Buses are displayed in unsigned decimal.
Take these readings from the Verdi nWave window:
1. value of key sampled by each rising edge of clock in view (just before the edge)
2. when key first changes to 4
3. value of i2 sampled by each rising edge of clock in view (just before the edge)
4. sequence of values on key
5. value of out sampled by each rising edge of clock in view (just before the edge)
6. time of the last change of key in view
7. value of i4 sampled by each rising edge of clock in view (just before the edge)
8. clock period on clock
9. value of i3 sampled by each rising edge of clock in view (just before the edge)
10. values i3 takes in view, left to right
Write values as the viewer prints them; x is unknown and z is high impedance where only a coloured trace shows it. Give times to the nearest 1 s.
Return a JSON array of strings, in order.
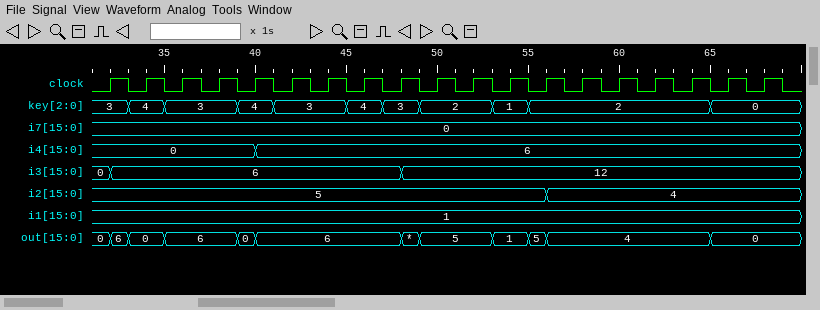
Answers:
["3, 4, 3, 3, 4, 3, 3, 4, 3, 2, 2, 1, 2, 2, 2, 2, 2, 0, 0", "33 s", "5, 5, 5, 5, 5, 5, 5, 5, 5, 5, 5, 5, 5, 4, 4, 4, 4, 4, 4", "3, 4, 3, 4, 3, 4, 3, 2, 1, 2, 0", "0, 0, 6, 6, 0, 6, 6, 6, 6, 5, 5, 1, 5, 4, 4, 4, 4, 0, 0", "65 s", "0, 0, 0, 0, 0, 6, 6, 6, 6, 6, 6, 6, 6, 6, 6, 6, 6, 6, 6", "2 s", "0, 6, 6, 6, 6, 6, 6, 6, 6, 12, 12, 12, 12, 12, 12, 12, 12, 12, 12", "0, 6, 12"]
